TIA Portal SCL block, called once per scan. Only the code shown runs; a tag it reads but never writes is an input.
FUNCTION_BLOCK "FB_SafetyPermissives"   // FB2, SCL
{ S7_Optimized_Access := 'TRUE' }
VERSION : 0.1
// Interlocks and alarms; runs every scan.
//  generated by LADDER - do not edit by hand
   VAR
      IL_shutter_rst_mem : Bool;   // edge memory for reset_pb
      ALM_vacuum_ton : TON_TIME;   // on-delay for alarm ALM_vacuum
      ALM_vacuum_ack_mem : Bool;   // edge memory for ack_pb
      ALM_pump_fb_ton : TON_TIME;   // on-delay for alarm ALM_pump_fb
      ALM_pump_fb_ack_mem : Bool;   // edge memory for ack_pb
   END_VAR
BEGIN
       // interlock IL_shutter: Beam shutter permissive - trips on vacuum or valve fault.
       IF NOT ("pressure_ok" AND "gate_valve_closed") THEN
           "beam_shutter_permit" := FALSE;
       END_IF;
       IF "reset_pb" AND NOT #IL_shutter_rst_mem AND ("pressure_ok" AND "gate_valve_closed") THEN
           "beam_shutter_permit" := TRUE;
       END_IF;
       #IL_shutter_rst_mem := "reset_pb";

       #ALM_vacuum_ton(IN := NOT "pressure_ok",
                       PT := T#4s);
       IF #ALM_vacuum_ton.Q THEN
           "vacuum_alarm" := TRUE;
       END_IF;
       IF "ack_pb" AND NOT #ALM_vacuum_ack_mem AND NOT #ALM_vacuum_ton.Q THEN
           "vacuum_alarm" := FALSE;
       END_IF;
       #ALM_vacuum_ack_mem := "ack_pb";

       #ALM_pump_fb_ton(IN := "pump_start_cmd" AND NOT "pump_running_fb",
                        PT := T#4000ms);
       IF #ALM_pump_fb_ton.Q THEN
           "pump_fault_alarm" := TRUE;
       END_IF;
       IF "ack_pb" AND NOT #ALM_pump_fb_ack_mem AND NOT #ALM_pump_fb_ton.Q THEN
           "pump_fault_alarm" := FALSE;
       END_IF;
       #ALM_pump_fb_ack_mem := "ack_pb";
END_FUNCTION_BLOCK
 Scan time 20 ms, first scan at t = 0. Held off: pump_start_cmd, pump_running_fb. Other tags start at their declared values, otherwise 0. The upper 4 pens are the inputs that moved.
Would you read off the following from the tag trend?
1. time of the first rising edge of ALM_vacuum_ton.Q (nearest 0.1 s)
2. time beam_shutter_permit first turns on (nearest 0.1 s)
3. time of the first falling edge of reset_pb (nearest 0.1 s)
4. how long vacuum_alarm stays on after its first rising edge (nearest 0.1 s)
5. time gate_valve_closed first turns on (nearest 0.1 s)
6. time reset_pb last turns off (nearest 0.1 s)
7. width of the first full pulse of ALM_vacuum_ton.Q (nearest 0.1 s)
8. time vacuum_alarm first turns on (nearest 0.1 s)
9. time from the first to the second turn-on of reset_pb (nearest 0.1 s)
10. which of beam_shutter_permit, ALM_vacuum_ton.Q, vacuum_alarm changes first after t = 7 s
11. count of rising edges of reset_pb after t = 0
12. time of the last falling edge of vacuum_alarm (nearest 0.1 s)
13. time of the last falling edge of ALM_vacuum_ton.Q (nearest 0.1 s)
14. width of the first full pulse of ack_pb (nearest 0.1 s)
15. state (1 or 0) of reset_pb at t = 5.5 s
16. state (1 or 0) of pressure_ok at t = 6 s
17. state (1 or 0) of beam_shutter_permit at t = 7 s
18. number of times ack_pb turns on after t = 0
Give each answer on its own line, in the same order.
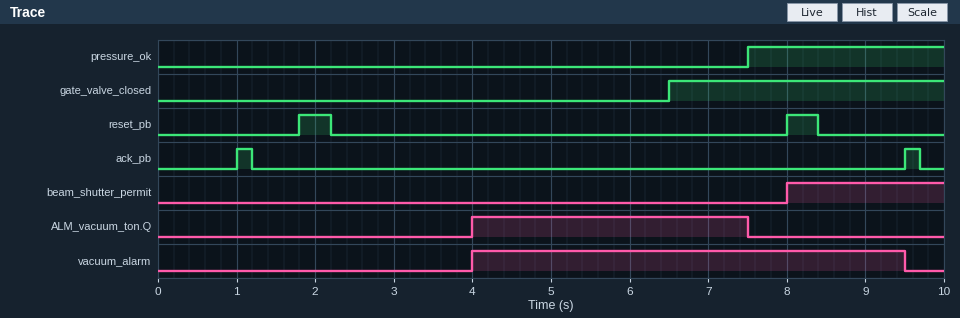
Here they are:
4.0 s
8.0 s
2.2 s
5.5 s
6.5 s
8.4 s
3.5 s
4.0 s
6.2 s
ALM_vacuum_ton.Q
2
9.5 s
7.5 s
0.2 s
0
0
0
2
